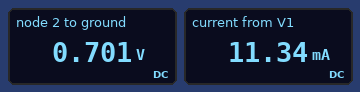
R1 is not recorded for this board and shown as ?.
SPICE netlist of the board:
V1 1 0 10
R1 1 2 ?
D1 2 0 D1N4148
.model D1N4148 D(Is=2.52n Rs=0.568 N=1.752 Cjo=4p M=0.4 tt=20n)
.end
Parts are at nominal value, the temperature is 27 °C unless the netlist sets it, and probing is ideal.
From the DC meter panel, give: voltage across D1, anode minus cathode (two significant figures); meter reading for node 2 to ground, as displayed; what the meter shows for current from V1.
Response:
700 mV
0.701 V
11.34 mA
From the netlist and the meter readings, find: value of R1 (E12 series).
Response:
820 Ω
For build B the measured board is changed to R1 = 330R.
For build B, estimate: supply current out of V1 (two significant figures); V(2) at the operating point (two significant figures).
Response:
28 mA
750 mV
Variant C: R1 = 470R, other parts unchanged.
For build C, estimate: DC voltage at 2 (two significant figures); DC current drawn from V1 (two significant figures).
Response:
730 mV
20 mA
